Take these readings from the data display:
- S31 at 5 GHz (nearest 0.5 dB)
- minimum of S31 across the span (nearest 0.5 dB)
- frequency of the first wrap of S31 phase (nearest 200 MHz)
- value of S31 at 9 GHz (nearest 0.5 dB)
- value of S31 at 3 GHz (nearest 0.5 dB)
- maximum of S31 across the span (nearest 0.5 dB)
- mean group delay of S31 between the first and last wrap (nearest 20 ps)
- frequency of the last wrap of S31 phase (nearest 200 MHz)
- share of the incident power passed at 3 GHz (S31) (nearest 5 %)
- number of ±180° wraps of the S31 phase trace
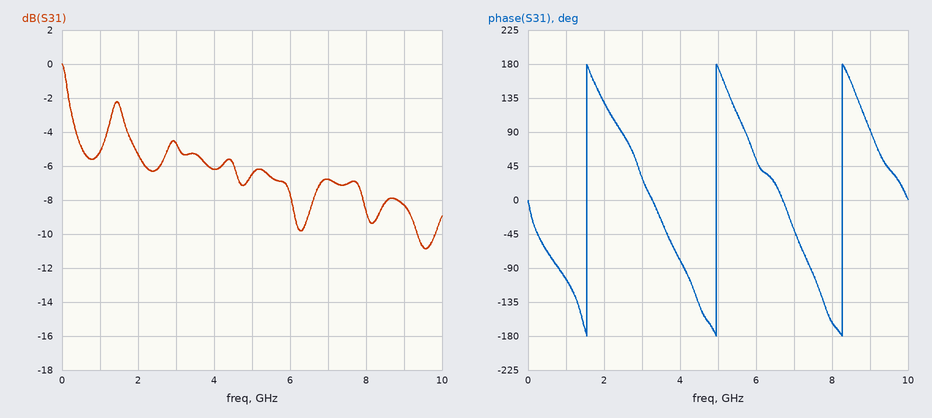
-6.5 dB
-11.0 dB
1.6 GHz
-8.5 dB
-4.5 dB
0.0 dB
300 ps
8.2 GHz
35 %
3
